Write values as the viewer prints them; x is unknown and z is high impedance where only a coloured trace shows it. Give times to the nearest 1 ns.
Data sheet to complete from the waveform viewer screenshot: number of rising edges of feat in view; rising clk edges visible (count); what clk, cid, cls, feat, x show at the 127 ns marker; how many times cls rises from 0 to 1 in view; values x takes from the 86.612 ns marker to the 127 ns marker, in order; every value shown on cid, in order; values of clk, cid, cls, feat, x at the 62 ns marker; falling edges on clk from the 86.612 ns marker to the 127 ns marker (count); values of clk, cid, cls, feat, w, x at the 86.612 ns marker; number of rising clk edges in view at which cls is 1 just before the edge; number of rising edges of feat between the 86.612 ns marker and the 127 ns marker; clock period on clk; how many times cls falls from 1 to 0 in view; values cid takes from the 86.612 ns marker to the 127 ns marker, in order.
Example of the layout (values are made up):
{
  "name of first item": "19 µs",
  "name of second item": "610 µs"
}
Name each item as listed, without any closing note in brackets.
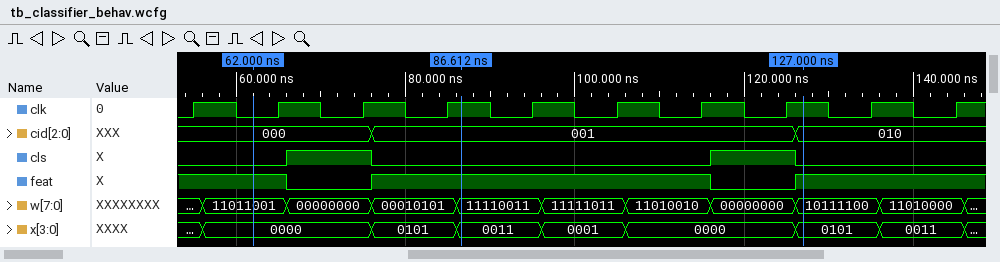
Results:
{
  "number of rising edges of feat in view": "2",
  "rising clk edges visible": "10",
  "what clk, cid, cls, feat, x show at the 127 ns marker": "clk=1, cid=010, cls=0, feat=1, x=0101",
  "how many times cls rises from 0 to 1 in view": "2",
  "values x takes from the 86.612 ns marker to the 127 ns marker, in order": "0011, 0001, 0000, 0101",
  "every value shown on cid, in order": "000, 001, 010",
  "values of clk, cid, cls, feat, x at the 62 ns marker": "clk=0, cid=000, cls=0, feat=1, x=0000",
  "falling edges on clk from the 86.612 ns marker to the 127 ns marker": "4",
  "values of clk, cid, cls, feat, w, x at the 86.612 ns marker": "clk=1, cid=001, cls=0, feat=1, w=11110011, x=0011",
  "number of rising clk edges in view at which cls is 1 just before the edge": "2",
  "number of rising edges of feat between the 86.612 ns marker and the 127 ns marker": "1",
  "clock period on clk": "10 ns",
  "how many times cls falls from 1 to 0 in view": "2",
  "values cid takes from the 86.612 ns marker to the 127 ns marker, in order": "001, 010"
}
